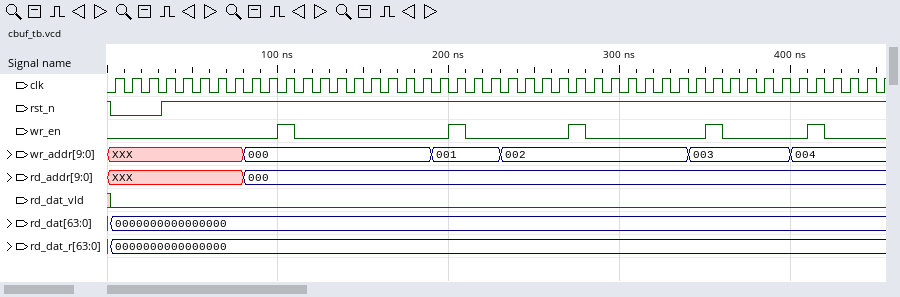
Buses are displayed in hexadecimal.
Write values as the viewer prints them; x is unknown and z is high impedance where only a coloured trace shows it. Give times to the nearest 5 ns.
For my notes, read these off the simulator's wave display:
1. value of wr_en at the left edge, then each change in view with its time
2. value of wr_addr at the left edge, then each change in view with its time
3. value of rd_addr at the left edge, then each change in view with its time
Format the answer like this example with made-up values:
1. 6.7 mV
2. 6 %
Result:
1. 0, 1 at 100 ns, 0 at 110 ns, 1 at 200 ns, 0 at 210 ns, 1 at 270 ns, 0 at 280 ns, 1 at 350 ns, 0 at 360 ns, 1 at 410 ns, 0 at 420 ns
2. XXX, 000 at 80 ns, 001 at 190 ns, 002 at 230 ns, 003 at 340 ns, 004 at 400 ns
3. XXX, 000 at 80 ns
